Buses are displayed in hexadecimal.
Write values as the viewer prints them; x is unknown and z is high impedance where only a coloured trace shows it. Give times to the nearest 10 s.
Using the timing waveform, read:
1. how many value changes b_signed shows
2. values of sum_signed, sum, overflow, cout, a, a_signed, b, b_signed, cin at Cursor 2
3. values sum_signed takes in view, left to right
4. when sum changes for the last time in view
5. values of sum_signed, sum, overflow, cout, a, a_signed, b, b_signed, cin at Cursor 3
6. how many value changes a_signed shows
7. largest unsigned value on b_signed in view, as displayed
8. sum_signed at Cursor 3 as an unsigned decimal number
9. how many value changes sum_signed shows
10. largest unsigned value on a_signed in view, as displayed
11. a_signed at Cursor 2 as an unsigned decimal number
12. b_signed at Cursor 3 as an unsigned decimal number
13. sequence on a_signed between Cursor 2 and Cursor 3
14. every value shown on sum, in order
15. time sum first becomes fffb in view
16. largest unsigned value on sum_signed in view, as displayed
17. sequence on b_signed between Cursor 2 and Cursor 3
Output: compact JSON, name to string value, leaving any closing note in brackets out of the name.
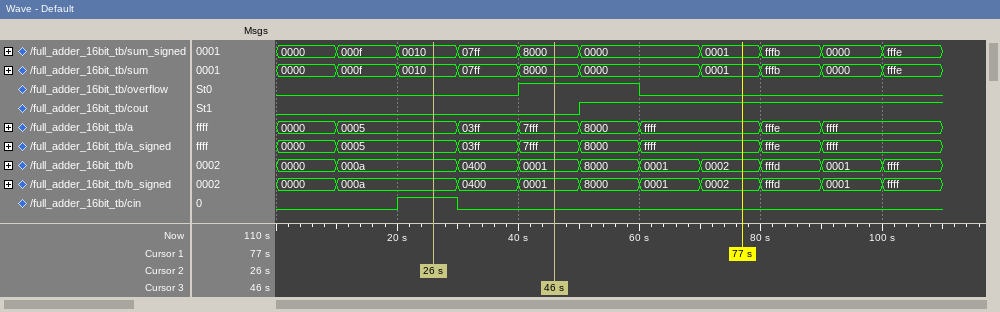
{"how many value changes b_signed shows": "9", "values of sum_signed, sum, overflow, cout, a, a_signed, b, b_signed, cin at Cursor 2": "sum_signed=0010, sum=0010, overflow=0, cout=0, a=0005, a_signed=0005, b=000a, b_signed=000a, cin=1", "values sum_signed takes in view, left to right": "0000, 000f, 0010, 07ff, 8000, 0000, 0001, fffb, 0000, fffe", "when sum changes for the last time in view": "100 s", "values of sum_signed, sum, overflow, cout, a, a_signed, b, b_signed, cin at Cursor 3": "sum_signed=8000, sum=8000, overflow=1, cout=0, a=7fff, a_signed=7fff, b=0001, b_signed=0001, cin=0", "how many value changes a_signed shows": "7", "largest unsigned value on b_signed in view, as displayed": "ffff", "sum_signed at Cursor 3 as an unsigned decimal number": "32768", "how many value changes sum_signed shows": "9", "largest unsigned value on a_signed in view, as displayed": "ffff", "a_signed at Cursor 2 as an unsigned decimal number": "5", "b_signed at Cursor 3 as an unsigned decimal number": "1", "sequence on a_signed between Cursor 2 and Cursor 3": "0005, 03ff, 7fff", "every value shown on sum, in order": "0000, 000f, 0010, 07ff, 8000, 0000, 0001, fffb, 0000, fffe", "time sum first becomes fffb in view": "80 s", "largest unsigned value on sum_signed in view, as displayed": "fffe", "sequence on b_signed between Cursor 2 and Cursor 3": "000a, 0400, 0001"}
